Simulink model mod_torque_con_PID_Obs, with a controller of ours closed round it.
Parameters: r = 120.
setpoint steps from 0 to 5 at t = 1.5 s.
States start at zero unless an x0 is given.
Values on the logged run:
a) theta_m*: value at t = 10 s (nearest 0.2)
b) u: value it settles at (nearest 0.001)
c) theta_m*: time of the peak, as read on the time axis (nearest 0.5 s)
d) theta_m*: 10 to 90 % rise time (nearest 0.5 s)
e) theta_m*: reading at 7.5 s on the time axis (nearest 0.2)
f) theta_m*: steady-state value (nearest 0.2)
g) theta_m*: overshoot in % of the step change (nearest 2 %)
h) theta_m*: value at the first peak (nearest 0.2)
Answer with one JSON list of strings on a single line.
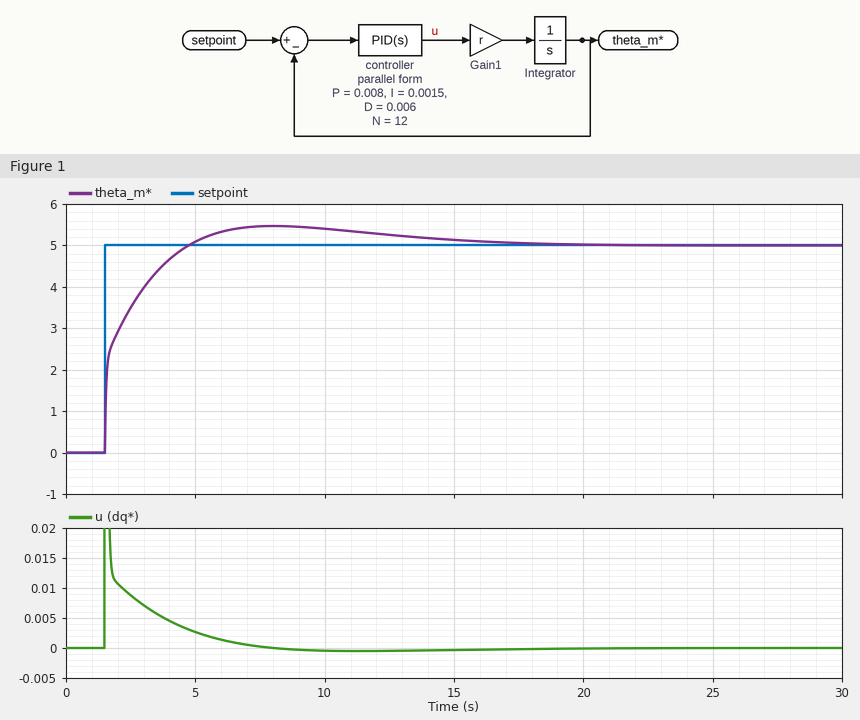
["5.4", "0.000", "8.0 s", "2.0 s", "5.4", "5.0", "10 %", "5.4"]
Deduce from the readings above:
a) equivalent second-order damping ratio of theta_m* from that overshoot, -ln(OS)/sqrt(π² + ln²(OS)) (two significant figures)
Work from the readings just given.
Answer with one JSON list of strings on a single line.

["0.59"]
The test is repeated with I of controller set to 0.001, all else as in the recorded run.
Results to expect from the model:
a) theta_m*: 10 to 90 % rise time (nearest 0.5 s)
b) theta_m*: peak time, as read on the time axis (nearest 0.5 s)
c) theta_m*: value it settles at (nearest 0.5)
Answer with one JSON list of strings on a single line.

["2.5 s", "9.0 s", "5.0"]
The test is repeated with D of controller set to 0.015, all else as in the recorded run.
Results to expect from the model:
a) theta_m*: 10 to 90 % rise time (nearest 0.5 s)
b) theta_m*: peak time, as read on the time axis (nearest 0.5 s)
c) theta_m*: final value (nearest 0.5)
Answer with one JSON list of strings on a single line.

["2.5 s", "10.5 s", "5.0"]
